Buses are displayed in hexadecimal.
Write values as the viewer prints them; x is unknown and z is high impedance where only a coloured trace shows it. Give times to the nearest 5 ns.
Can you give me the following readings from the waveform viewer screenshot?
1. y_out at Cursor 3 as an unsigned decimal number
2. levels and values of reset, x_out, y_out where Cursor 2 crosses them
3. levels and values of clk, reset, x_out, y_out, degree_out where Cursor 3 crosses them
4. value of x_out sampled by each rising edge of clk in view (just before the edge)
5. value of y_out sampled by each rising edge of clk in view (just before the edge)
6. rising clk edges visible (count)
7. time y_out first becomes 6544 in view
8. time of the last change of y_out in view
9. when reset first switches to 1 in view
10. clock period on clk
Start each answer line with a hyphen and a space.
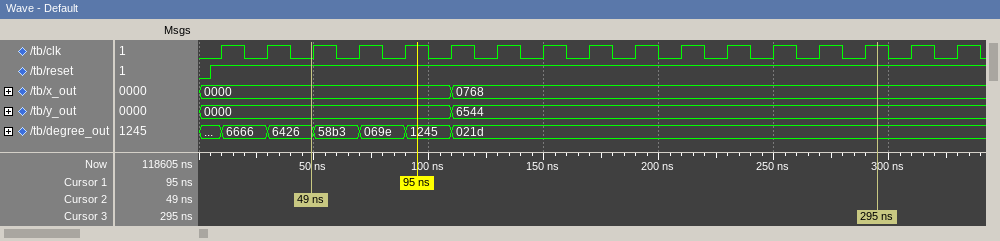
- 25924
- reset=1, x_out=0000, y_out=0000
- clk=1, reset=1, x_out=0768, y_out=6544, degree_out=021d
- 0000, 0000, 0000, 0000, 0000, 0000, 0768, 0768, 0768, 0768, 0768, 0768, 0768, 0768, 0768, 0768, 0768
- 0000, 0000, 0000, 0000, 0000, 0000, 6544, 6544, 6544, 6544, 6544, 6544, 6544, 6544, 6544, 6544, 6544
- 17
- 110 ns
- 110 ns
- 5 ns
- 20 ns
